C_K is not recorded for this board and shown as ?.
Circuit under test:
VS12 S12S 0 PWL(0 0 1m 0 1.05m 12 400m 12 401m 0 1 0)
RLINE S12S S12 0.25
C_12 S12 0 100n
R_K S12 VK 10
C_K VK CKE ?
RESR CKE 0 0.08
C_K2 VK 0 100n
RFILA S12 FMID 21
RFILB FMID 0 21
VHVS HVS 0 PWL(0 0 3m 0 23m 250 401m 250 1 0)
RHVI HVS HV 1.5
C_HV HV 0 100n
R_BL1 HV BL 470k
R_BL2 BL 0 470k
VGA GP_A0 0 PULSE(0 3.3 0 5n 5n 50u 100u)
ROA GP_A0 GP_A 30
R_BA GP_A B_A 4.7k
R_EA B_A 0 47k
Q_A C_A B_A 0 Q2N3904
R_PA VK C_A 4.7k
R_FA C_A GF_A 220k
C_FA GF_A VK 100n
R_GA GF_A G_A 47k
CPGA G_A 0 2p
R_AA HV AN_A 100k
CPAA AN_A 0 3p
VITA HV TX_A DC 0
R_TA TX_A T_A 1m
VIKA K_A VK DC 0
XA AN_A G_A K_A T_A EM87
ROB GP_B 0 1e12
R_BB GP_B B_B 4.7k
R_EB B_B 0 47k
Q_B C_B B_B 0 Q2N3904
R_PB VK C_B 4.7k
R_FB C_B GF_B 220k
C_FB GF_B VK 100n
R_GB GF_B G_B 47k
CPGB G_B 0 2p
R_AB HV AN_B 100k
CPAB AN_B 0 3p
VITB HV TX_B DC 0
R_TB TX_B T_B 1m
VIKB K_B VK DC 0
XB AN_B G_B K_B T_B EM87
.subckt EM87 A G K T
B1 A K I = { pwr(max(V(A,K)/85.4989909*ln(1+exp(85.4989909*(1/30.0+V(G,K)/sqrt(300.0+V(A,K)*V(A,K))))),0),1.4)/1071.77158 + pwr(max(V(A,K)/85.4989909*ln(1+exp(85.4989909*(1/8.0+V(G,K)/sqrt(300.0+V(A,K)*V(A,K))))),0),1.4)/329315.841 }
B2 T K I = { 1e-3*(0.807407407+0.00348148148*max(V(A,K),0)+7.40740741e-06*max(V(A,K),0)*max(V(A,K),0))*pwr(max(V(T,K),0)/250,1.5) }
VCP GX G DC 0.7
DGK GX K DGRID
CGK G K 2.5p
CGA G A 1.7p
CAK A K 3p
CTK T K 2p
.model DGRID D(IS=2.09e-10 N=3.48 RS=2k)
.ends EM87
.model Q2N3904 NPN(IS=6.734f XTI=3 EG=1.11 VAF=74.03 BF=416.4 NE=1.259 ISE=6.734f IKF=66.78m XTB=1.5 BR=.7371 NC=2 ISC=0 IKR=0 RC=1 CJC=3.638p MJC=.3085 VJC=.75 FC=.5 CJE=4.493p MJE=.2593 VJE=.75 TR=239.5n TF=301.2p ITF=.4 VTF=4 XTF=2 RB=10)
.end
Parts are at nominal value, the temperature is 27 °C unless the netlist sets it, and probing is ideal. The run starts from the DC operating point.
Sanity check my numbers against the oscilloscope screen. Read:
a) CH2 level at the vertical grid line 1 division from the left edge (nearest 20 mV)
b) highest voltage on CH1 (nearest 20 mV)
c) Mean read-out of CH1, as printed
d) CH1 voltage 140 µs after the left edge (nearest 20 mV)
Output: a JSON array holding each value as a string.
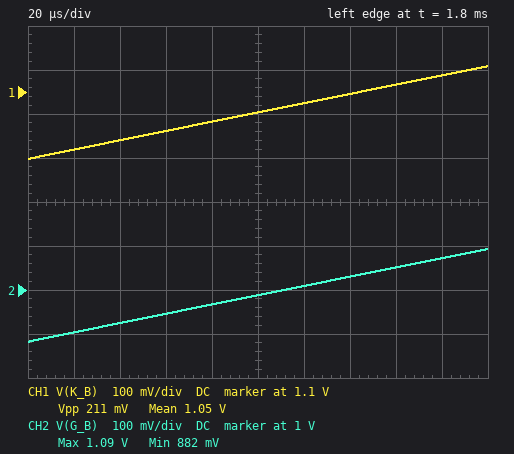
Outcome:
["900 mV", "1.16 V", "1.05 V", "1.10 V"]
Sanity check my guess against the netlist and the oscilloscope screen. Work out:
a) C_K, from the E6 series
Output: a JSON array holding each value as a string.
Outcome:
["1 mF"]
